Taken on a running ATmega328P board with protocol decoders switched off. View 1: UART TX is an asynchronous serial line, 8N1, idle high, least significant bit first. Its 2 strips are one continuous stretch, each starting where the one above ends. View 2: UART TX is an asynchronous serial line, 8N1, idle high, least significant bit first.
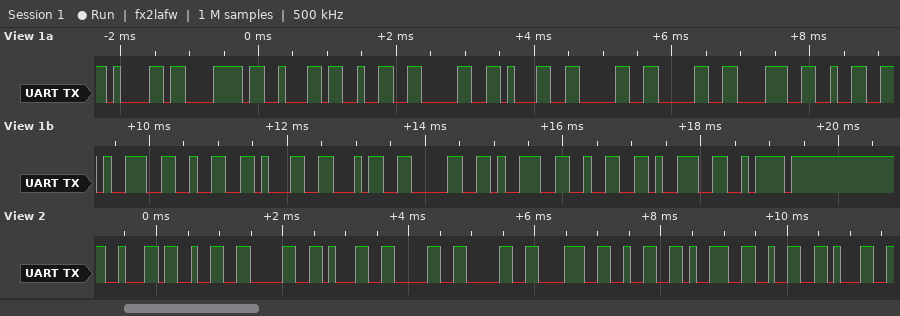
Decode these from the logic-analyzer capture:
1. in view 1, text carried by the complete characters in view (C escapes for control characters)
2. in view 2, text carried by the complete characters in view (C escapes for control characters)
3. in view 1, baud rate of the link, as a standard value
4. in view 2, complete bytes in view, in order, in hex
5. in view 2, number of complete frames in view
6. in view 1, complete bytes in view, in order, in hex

"axb201008292140929z"
"b2010082921"
9600 baud
62 32 30 31 30 30 38 32 39 32 31
11
61 78 62 32 30 31 30 30 38 32 39 32 31 34 30 39 32 39 7A
